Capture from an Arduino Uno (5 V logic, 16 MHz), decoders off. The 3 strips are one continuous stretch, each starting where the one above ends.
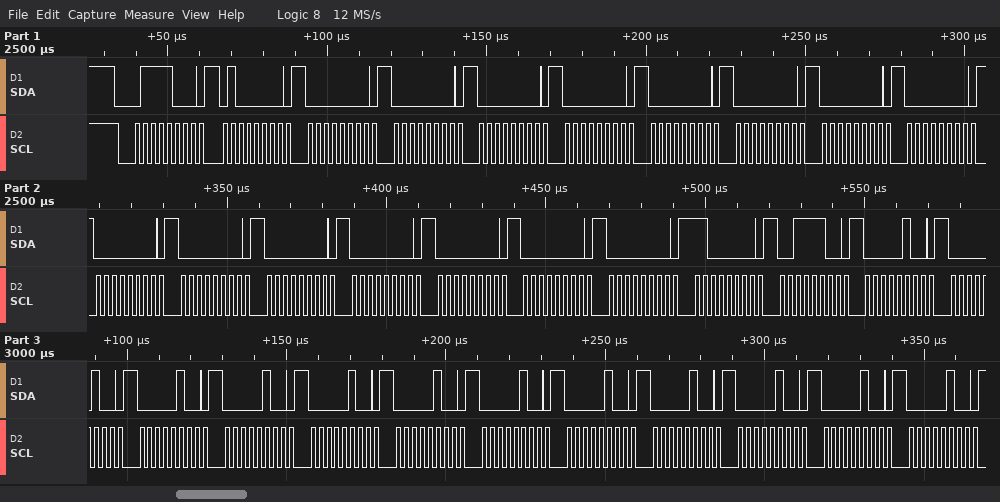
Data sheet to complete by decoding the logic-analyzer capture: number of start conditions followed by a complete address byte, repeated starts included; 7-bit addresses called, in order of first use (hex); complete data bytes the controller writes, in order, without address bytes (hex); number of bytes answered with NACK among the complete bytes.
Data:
1
0x3C
40 00 00 00 00 00 00 00 00 00 00 00 00 00 00 00 C0 3C 04 04 04 04 04 04 04 04 04 04 04 04
0
